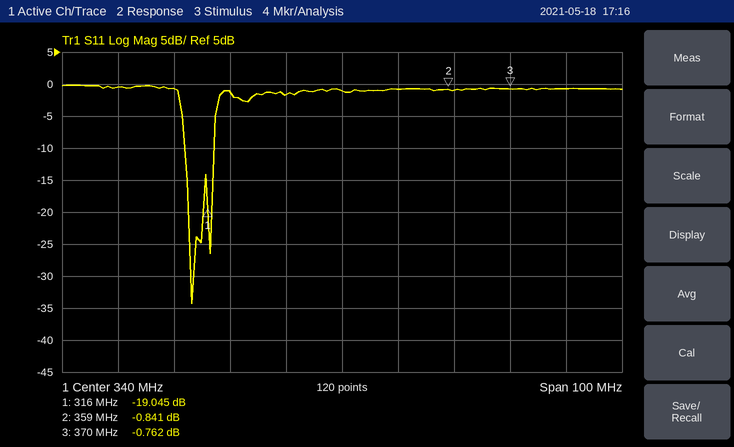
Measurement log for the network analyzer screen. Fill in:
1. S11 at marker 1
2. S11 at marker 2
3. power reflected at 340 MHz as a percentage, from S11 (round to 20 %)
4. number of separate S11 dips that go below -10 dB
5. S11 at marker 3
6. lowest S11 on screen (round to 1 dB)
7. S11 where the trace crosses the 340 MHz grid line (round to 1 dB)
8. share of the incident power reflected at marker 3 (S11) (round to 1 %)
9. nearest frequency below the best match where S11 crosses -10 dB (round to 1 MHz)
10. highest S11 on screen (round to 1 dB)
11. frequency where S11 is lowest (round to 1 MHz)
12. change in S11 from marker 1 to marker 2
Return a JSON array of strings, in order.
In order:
["-19.045 dB", "-0.841 dB", "80 %", "2", "-0.762 dB", "-34 dB", "-1 dB", "84 %", "312 MHz", "0 dB", "313 MHz", "18.204 dB"]
